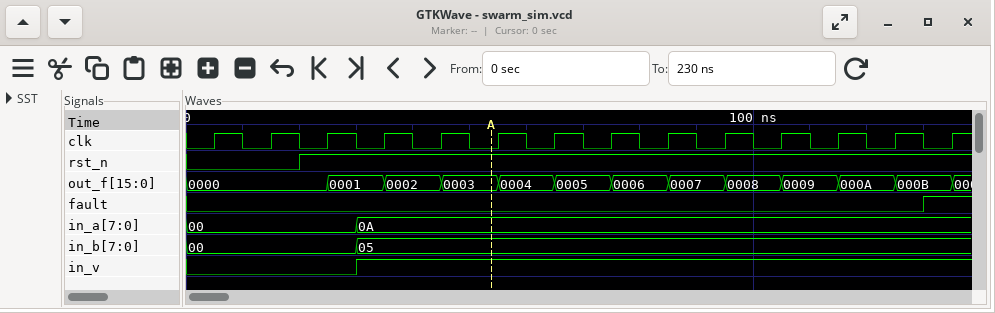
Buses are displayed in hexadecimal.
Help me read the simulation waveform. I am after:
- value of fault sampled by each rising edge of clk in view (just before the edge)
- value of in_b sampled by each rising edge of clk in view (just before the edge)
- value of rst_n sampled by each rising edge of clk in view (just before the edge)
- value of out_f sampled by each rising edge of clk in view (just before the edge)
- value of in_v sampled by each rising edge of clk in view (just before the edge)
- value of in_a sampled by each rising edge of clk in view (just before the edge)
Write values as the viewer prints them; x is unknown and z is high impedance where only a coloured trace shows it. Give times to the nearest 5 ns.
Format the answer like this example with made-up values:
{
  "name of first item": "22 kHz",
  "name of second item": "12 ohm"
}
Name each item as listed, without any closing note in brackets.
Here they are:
{
  "value of fault sampled by each rising edge of clk in view": "0 0 0 0 0 0 0 0 0 0 0 0 0 1",
  "value of in_b sampled by each rising edge of clk in view": "00, 00, 00, 05, 05, 05, 05, 05, 05, 05, 05, 05, 05, 05",
  "value of rst_n sampled by each rising edge of clk in view": "0 0 1 1 1 1 1 1 1 1 1 1 1 1",
  "value of out_f sampled by each rising edge of clk in view": "0000, 0000, 0000, 0001, 0002, 0003, 0004, 0005, 0006, 0007, 0008, 0009, 000A, 000B",
  "value of in_v sampled by each rising edge of clk in view": "0 0 0 1 1 1 1 1 1 1 1 1 1 1",
  "value of in_a sampled by each rising edge of clk in view": "00, 00, 00, 0A, 0A, 0A, 0A, 0A, 0A, 0A, 0A, 0A, 0A, 0A"
}
